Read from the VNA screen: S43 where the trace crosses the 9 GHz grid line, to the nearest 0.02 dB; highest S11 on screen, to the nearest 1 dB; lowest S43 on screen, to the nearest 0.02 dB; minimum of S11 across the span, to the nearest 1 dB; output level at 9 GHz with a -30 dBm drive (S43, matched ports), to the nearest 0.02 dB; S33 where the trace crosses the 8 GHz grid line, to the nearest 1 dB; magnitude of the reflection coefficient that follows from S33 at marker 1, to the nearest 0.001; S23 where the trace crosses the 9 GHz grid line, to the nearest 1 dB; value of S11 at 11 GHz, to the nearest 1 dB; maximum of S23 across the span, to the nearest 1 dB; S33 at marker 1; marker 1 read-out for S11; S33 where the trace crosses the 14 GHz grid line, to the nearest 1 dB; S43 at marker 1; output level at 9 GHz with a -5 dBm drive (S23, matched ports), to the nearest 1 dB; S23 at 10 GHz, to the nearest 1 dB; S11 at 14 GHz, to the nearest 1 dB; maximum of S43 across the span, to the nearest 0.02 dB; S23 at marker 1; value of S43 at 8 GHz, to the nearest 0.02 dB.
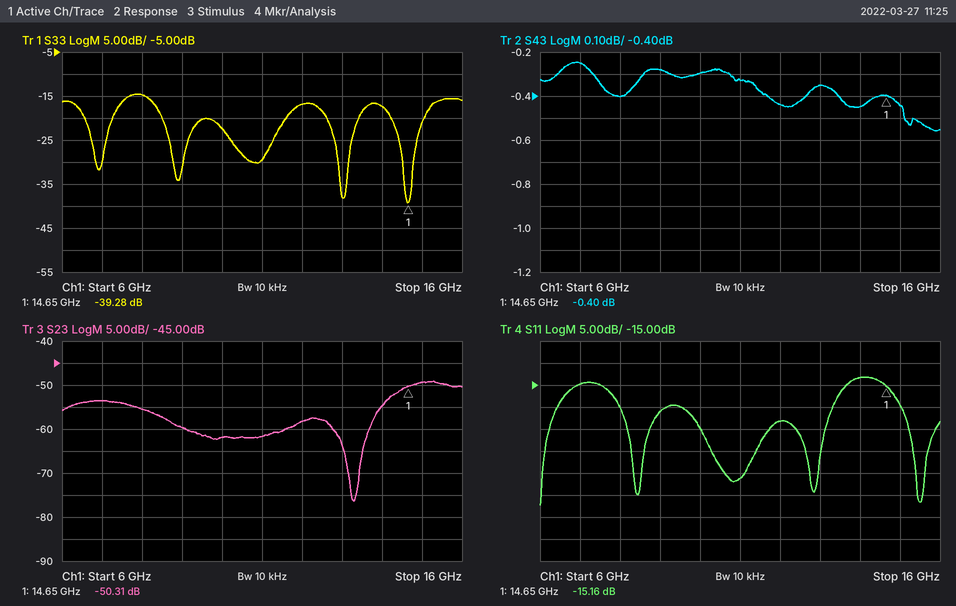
-0.28 dB
-13 dB
-0.56 dB
-42 dB
-30.28 dBm
-15 dB
0.011
-60 dB
-36 dB
-49 dB
-39.28 dB
-15.16 dB
-17 dB
-0.40 dB
-65 dBm
-62 dB
-13 dB
-0.24 dB
-50.31 dB
-0.40 dB
